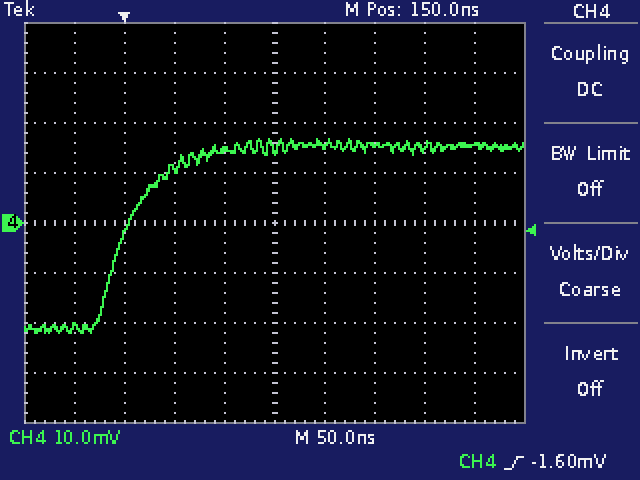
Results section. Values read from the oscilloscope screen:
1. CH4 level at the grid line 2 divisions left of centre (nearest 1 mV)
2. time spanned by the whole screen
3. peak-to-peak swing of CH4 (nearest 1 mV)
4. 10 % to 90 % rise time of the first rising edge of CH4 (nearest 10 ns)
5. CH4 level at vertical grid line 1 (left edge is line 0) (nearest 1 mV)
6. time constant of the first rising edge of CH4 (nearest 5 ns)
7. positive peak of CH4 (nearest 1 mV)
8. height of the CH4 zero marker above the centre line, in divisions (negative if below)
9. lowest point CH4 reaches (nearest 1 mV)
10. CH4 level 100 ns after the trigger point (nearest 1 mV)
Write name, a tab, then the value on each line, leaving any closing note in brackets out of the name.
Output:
CH4 level at the grid line 2 divisions left of centre	11 mV
time spanned by the whole screen	500 ns
peak-to-peak swing of CH4	39 mV
10 % to 90 % rise time of the first rising edge of CH4	80 ns
CH4 level at vertical grid line 1 (left edge is line 0)	-21 mV
time constant of the first rising edge of CH4	35 ns
positive peak of CH4	17 mV
height of the CH4 zero marker above the centre line, in divisions	0.0 div
lowest point CH4 reaches	-22 mV
CH4 level 100 ns after the trigger point	15 mV
